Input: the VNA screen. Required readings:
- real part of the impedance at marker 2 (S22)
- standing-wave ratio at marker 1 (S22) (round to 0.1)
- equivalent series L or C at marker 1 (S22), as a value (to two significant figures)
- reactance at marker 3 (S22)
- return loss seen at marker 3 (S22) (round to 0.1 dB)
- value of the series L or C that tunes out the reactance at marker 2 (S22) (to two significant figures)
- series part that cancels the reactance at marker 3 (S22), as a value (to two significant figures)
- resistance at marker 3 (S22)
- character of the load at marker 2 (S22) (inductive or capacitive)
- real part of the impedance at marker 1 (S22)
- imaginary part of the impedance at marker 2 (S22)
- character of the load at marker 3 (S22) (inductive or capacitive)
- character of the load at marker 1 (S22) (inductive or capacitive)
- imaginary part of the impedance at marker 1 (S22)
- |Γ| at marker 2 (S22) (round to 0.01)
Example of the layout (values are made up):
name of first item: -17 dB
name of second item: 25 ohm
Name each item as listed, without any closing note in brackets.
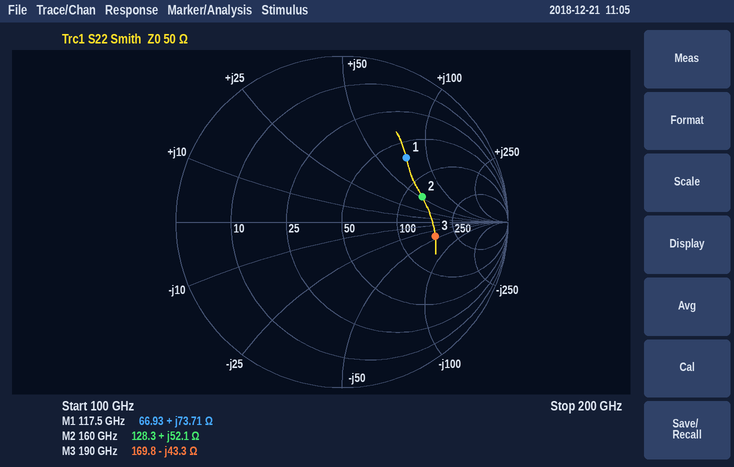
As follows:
real part of the impedance at marker 2: 128.3 Ω
standing-wave ratio at marker 1 (S22): 3.4
equivalent series L or C at marker 1 (S22), as a value: 100 pH
reactance at marker 3: -43.3 Ω
return loss seen at marker 3 (S22): 4.9 dB
value of the series L or C that tunes out the reactance at marker 2 (S22): 19 fF
series part that cancels the reactance at marker 3 (S22), as a value: 36 pH
resistance at marker 3: 169.8 Ω
character of the load at marker 2 (S22): inductive
real part of the impedance at marker 1: 66.93 Ω
imaginary part of the impedance at marker 2: +52.1 Ω
character of the load at marker 3 (S22): capacitive
character of the load at marker 1 (S22): inductive
imaginary part of the impedance at marker 1: +73.71 Ω
|Γ| at marker 2 (S22): 0.51
